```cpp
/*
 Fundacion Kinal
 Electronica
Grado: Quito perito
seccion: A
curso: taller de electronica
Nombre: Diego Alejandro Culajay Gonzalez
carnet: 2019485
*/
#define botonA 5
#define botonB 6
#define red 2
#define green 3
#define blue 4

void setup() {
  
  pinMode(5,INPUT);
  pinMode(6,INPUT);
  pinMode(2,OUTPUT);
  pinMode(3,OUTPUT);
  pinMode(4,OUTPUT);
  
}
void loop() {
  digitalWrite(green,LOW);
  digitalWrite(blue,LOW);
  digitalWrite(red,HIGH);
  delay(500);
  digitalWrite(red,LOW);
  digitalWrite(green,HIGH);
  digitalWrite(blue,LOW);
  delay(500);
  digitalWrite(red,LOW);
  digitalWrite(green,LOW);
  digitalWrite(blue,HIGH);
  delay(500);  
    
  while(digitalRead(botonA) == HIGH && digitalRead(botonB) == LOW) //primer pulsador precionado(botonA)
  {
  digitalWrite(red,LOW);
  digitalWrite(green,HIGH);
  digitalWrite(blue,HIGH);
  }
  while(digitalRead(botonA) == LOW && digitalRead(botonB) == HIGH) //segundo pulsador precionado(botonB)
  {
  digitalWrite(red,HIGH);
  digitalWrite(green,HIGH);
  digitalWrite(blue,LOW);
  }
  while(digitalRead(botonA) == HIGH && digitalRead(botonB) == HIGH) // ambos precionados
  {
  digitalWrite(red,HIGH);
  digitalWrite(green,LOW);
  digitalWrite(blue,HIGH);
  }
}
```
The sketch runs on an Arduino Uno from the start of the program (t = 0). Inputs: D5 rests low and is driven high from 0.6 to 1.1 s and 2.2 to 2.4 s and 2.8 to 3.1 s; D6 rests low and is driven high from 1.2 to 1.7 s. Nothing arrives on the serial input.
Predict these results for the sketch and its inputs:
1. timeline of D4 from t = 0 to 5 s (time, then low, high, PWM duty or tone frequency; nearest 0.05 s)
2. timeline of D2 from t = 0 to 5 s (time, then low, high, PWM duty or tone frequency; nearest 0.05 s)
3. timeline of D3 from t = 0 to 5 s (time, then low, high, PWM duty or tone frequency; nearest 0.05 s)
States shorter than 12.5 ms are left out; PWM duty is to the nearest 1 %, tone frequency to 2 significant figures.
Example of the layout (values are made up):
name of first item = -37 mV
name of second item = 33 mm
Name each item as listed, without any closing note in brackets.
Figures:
timeline of D4 from t = 0 to 5 s = 0 s low; 1 s high; 1.5 s low; 2.7 s high; 3.2 s low; 4.2 s high; 4.7 s low
timeline of D2 from t = 0 to 5 s = 0 s high; 0.5 s low; 1.5 s high; 2.2 s low; 3.2 s high; 3.7 s low; 4.7 s high
timeline of D3 from t = 0 to 5 s = 0 s low; 0.5 s high; 1 s low; 1.5 s high; 1.7 s low; 2.2 s high; 2.7 s low; 3.7 s high; 4.2 s low
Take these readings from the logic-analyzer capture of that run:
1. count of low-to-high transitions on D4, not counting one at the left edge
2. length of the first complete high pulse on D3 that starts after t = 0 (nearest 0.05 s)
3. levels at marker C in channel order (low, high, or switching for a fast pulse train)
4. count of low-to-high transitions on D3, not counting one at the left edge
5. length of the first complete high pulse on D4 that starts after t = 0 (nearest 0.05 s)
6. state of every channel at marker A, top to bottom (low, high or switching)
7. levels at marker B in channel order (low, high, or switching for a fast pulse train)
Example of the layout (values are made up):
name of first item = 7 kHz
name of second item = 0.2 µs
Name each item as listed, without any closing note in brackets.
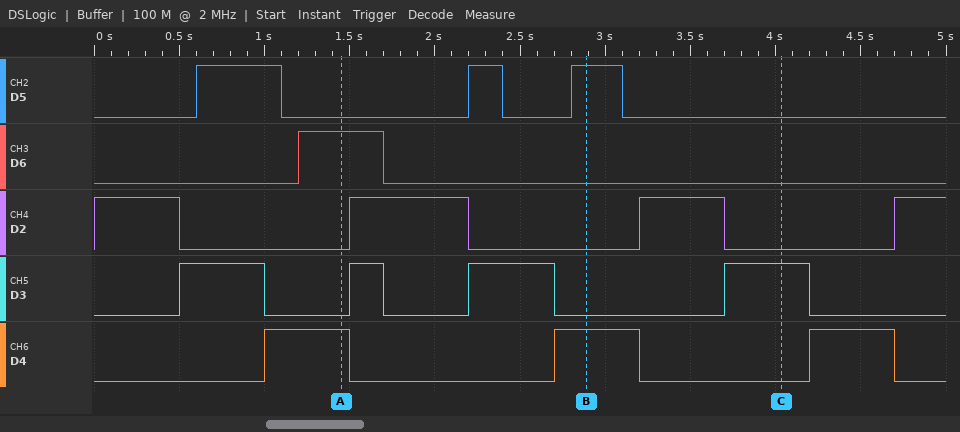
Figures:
count of low-to-high transitions on D4, not counting one at the left edge = 3
length of the first complete high pulse on D3 that starts after t = 0 = 0.50 s
levels at marker C in channel order = D5 low, D6 low, D2 low, D3 high, D4 low
count of low-to-high transitions on D3, not counting one at the left edge = 4
length of the first complete high pulse on D4 that starts after t = 0 = 0.50 s
state of every channel at marker A, top to bottom = D5 low, D6 high, D2 low, D3 low, D4 high
levels at marker B in channel order = D5 high, D6 low, D2 low, D3 low, D4 high
